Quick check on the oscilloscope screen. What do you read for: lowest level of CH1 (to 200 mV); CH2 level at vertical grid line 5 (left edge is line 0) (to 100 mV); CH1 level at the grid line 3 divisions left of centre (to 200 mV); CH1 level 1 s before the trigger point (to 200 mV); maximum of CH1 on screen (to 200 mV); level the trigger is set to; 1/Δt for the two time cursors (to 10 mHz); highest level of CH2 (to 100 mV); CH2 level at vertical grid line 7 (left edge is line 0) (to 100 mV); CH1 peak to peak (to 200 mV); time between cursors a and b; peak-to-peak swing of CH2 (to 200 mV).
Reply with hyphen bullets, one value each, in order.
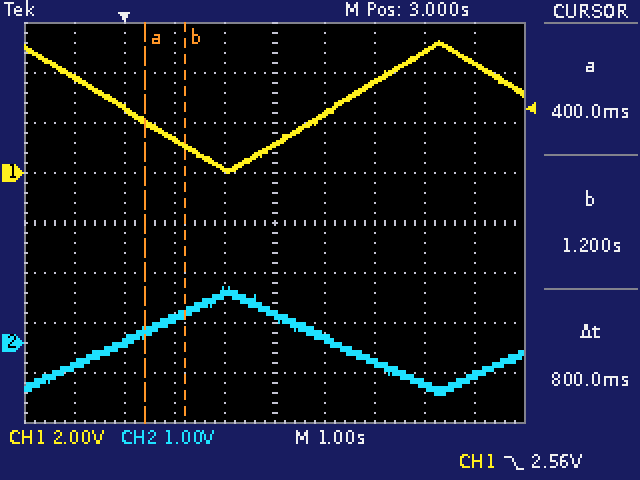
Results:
- 0.0 V
- 600 mV
- 2.6 V
- 3.8 V
- 5.2 V
- 2.56 V
- 1.25 Hz
- 1.1 V
- -400 mV
- 5.2 V
- 800 ms
- 2.2 V
